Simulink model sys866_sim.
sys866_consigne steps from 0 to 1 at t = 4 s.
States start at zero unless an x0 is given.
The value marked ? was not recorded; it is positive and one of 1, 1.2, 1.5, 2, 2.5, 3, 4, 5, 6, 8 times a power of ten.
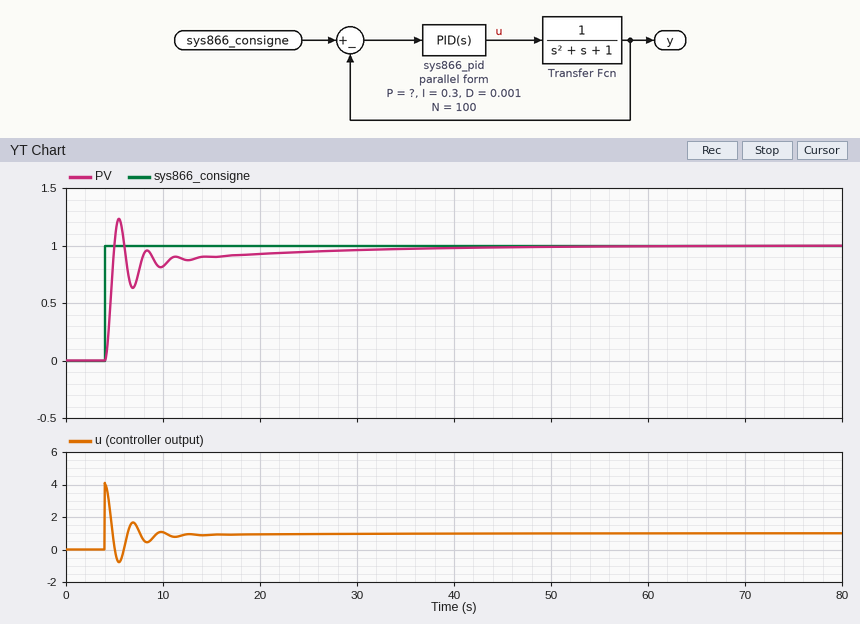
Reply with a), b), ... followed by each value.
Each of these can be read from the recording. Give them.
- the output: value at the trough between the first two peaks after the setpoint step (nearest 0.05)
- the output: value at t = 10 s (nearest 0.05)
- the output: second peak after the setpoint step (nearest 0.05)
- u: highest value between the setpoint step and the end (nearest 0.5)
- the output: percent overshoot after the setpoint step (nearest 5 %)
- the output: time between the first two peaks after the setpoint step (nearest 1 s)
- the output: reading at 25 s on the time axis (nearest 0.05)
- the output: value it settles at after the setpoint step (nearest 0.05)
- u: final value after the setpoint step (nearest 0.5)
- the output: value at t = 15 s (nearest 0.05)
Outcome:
a) 0.65
b) 0.80
c) 0.95
d) 4.0
e) 25 %
f) 3 s
g) 0.95
h) 1.00
i) 1.0
j) 0.90
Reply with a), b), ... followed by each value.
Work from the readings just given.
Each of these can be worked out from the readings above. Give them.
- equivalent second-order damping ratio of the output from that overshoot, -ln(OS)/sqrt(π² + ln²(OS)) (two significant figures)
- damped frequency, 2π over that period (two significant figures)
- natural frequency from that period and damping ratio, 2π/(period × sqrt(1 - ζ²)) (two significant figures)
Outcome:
a) 0.40
b) 2.1 rad/s
c) 2.3 rad/s
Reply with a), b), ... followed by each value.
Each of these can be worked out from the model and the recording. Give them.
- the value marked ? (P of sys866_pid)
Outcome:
a) 4
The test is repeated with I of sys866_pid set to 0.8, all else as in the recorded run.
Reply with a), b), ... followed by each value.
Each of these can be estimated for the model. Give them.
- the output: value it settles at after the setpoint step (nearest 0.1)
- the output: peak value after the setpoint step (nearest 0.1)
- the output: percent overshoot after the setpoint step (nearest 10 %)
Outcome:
a) 1.0
b) 1.3
c) 30 %
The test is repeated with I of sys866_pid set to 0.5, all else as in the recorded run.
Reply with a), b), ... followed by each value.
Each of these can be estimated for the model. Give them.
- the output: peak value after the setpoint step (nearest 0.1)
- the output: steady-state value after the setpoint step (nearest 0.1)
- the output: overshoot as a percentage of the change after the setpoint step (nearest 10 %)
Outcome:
a) 1.3
b) 1.0
c) 30 %
